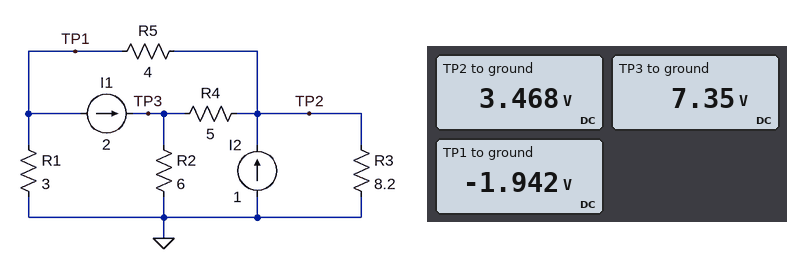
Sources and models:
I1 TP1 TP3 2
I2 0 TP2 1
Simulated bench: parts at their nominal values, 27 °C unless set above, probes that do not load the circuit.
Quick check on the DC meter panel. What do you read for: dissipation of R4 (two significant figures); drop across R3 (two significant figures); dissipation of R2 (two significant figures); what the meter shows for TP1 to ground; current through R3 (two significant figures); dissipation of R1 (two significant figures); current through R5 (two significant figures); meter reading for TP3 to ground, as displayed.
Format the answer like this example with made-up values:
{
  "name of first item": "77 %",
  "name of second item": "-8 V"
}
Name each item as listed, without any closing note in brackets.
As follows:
{
  "dissipation of R4": "3.0 W",
  "drop across R3": "3.5 V",
  "dissipation of R2": "9.0 W",
  "what the meter shows for TP1 to ground": "-1.942 V",
  "current through R3": "420 mA",
  "dissipation of R1": "1.3 W",
  "current through R5": "1.4 A",
  "meter reading for TP3 to ground, as displayed": "7.35 V"
}
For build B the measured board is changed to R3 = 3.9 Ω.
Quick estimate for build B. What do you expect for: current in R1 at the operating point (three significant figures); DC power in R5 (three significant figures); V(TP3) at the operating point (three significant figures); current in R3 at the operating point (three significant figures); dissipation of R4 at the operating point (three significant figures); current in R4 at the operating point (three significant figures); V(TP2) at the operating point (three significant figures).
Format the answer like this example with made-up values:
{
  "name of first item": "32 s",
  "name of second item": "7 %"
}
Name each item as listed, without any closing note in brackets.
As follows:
{
  "current in R1 at the operating point": "783 mA",
  "DC power in R5": "5.92 W",
  "V(TP3) at the operating point": "6.83 V",
  "current in R3 at the operating point": "645 mA",
  "dissipation of R4 at the operating point": "3.72 W",
  "current in R4 at the operating point": "862 mA",
  "V(TP2) at the operating point": "2.52 V"
}
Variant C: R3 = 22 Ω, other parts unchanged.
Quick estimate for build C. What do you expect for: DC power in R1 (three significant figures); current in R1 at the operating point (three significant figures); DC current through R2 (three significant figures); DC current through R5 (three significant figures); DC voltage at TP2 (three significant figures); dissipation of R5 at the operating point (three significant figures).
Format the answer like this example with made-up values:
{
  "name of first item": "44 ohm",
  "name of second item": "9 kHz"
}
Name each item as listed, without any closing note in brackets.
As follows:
{
  "DC power in R1": "785 mW",
  "current in R1 at the operating point": "512 mA",
  "DC current through R2": "1.31 A",
  "DC current through R5": "1.49 A",
  "DC voltage at TP2": "4.42 V",
  "dissipation of R5 at the operating point": "8.86 W"
}
